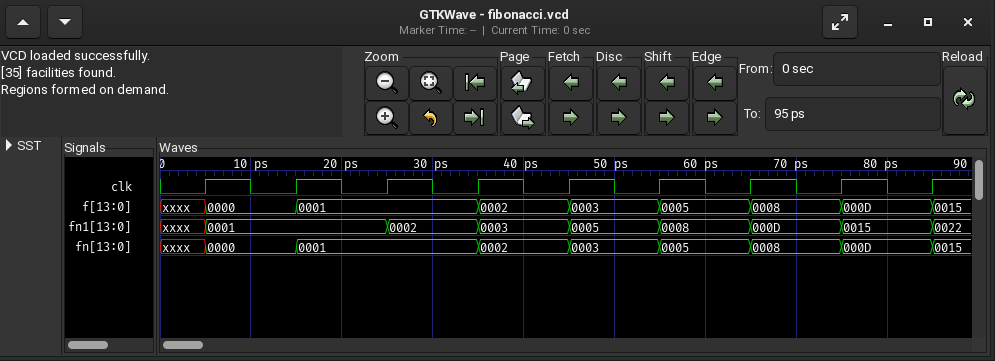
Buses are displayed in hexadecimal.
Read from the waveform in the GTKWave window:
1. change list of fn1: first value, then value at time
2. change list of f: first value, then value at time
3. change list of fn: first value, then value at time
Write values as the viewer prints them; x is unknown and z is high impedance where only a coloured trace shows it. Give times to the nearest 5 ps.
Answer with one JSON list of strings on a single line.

["xxxx, 0001 at 5 ps, 0002 at 25 ps, 0003 at 35 ps, 0005 at 45 ps, 0008 at 55 ps, 000D at 65 ps, 0015 at 75 ps, 0022 at 85 ps", "xxxx, 0000 at 5 ps, 0001 at 15 ps, 0002 at 35 ps, 0003 at 45 ps, 0005 at 55 ps, 0008 at 65 ps, 000D at 75 ps, 0015 at 85 ps", "xxxx, 0000 at 5 ps, 0001 at 15 ps, 0002 at 35 ps, 0003 at 45 ps, 0005 at 55 ps, 0008 at 65 ps, 000D at 75 ps, 0015 at 85 ps"]
